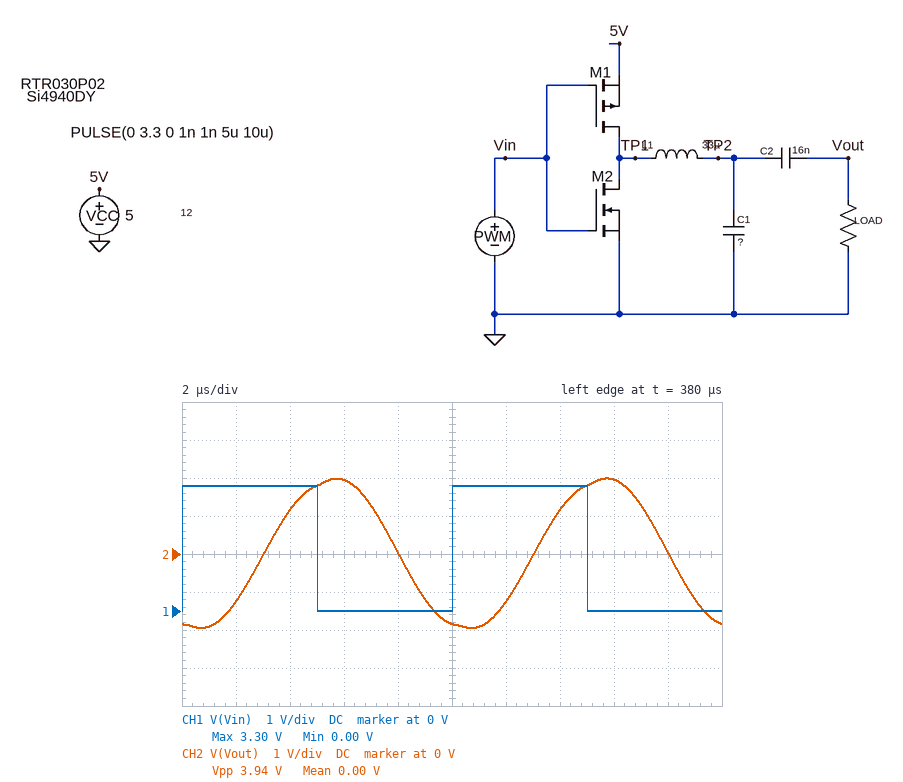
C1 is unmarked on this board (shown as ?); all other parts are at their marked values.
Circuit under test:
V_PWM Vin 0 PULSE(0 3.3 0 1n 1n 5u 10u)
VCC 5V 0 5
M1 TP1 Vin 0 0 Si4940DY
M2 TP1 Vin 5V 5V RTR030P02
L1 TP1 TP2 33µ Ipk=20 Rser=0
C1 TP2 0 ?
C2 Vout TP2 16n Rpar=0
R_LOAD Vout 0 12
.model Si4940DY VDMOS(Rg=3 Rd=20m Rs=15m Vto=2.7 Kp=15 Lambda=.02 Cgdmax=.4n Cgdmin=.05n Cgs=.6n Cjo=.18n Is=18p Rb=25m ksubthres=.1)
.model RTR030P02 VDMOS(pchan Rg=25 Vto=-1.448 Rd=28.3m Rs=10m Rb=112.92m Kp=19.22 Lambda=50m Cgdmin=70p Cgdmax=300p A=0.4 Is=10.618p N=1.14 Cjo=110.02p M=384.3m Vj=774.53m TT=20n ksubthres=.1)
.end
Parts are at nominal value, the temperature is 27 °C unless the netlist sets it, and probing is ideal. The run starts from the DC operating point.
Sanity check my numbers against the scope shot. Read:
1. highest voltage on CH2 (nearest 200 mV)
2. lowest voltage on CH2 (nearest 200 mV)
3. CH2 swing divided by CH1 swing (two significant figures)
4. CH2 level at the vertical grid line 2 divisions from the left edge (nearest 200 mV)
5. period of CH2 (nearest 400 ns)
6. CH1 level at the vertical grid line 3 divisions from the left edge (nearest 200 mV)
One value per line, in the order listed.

2.0 V
-2.0 V
1.2
1.2 V
10.0 µs
0 V
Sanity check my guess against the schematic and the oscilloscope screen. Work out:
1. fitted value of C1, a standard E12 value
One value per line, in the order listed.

47 nF
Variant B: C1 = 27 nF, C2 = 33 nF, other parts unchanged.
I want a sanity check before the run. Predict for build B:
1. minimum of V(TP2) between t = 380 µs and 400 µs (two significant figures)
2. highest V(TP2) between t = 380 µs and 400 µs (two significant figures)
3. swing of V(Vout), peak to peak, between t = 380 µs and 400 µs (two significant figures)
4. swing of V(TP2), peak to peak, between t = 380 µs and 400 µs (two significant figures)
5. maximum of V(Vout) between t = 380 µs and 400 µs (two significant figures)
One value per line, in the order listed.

-9.0 V
14 V
5.8 V
23 V
2.9 V
